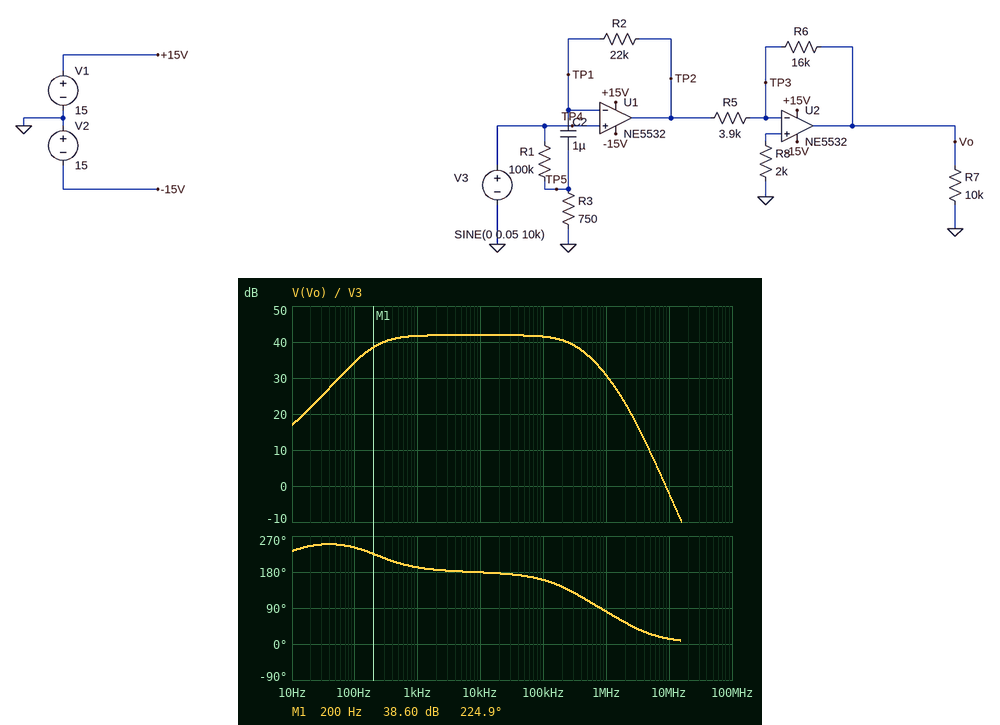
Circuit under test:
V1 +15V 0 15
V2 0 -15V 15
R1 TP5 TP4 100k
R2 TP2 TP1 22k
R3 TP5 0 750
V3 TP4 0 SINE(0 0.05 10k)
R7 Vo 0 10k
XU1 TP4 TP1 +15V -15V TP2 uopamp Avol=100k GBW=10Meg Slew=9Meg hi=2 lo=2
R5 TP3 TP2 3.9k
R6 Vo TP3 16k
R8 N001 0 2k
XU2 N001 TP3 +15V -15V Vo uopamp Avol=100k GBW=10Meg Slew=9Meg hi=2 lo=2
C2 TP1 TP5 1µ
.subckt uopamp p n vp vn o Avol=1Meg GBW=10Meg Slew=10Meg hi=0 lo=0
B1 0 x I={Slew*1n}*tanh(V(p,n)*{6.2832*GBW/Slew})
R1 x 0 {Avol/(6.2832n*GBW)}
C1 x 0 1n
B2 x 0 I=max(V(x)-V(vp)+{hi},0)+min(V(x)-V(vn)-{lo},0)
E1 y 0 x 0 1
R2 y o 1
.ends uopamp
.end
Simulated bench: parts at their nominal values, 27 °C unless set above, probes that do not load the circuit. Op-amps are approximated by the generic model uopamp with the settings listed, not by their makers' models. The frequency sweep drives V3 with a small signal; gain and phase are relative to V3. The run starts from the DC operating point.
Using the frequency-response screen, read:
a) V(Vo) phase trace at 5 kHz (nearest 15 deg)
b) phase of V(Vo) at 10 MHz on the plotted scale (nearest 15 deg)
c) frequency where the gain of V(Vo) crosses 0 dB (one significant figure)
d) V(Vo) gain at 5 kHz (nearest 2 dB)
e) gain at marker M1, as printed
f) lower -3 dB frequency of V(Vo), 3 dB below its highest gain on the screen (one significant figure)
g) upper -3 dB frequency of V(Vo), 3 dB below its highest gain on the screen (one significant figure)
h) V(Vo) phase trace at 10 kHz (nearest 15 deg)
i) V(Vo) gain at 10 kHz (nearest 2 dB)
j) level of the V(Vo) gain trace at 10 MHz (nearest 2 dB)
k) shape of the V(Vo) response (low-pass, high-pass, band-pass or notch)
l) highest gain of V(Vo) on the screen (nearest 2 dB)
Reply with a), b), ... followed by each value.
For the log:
a) 180 deg
b) 15 deg
c) 9 MHz
d) 42 dB
e) 38.60 dB
f) 200 Hz
g) 300 kHz
h) 180 deg
i) 42 dB
j) -2 dB
k) band-pass
l) 42 dB
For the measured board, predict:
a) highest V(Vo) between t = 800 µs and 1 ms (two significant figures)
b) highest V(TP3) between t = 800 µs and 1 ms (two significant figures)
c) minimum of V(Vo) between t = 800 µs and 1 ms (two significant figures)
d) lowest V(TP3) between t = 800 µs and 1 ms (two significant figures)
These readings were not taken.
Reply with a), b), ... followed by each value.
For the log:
a) 6.3 V
b) 6.2 mV
c) -6.2 V
d) -6.2 mV
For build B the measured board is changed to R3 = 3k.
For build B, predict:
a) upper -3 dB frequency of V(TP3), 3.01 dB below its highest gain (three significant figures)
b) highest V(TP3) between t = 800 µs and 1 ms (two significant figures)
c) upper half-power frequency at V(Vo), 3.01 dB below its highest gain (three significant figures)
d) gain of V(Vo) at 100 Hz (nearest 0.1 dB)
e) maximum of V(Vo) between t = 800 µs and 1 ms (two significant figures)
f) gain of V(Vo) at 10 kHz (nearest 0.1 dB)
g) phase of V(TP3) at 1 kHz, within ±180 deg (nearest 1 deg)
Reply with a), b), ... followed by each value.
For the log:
a) 3.74 MHz
b) 1.7 mV
c) 930 kHz
d) 29.6 dB
e) 1.7 V
f) 30.7 dB
g) 87 deg
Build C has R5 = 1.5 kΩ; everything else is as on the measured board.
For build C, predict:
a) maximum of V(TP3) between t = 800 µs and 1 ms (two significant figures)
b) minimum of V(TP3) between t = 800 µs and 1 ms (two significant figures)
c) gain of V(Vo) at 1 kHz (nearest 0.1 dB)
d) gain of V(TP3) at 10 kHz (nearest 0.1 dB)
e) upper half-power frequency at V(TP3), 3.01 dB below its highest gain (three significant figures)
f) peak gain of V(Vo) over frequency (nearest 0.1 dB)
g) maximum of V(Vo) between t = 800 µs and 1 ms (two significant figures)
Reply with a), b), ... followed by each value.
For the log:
a) 260 mV
b) -280 mV
c) 50.0 dB
d) -9.8 dB
e) 1.39 MHz
f) 50.2 dB
g) 13 V
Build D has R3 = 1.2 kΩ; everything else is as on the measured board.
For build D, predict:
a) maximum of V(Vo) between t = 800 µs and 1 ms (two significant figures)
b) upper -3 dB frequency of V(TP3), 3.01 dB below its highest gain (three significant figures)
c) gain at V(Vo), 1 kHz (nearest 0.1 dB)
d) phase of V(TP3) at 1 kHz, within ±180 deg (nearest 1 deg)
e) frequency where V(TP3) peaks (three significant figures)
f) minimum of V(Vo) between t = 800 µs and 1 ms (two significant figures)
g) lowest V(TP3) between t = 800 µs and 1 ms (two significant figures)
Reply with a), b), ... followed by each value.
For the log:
a) 4.0 V
b) 2.83 MHz
c) 37.9 dB
d) 91 deg
e) 1.00 MHz
f) -3.9 V
g) -4.0 mV
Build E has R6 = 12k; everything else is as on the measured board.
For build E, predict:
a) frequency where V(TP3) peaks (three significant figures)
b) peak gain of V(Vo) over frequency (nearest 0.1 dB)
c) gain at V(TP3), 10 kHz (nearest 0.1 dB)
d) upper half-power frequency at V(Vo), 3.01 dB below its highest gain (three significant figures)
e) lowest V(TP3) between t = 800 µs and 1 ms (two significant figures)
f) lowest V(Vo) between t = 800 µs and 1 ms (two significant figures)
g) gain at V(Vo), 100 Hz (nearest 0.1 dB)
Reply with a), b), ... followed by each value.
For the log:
a) 896 kHz
b) 39.4 dB
c) -20.6 dB
d) 322 kHz
e) -4.7 mV
f) -4.6 V
g) 32.0 dB
